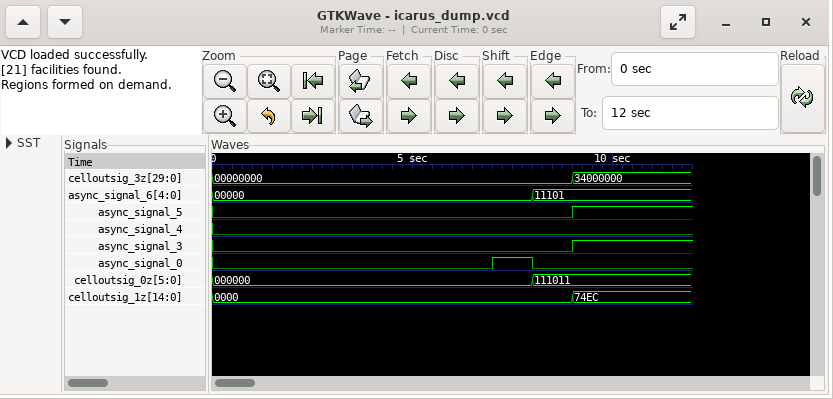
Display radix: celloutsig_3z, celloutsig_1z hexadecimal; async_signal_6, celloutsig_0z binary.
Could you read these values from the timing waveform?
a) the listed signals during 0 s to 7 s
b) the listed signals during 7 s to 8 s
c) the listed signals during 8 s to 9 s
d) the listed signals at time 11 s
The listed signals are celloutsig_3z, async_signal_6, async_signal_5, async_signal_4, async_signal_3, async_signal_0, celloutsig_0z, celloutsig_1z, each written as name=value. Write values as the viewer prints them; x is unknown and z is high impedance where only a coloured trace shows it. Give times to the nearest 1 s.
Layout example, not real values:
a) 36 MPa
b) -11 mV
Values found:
a) celloutsig_3z=00000000, async_signal_6=00000, async_signal_5=0, async_signal_4=0, async_signal_3=0, async_signal_0=0, celloutsig_0z=000000, celloutsig_1z=0000
b) celloutsig_3z=00000000, async_signal_6=00000, async_signal_5=0, async_signal_4=0, async_signal_3=0, async_signal_0=1, celloutsig_0z=000000, celloutsig_1z=0000
c) celloutsig_3z=00000000, async_signal_6=11101, async_signal_5=0, async_signal_4=0, async_signal_3=0, async_signal_0=0, celloutsig_0z=111011, celloutsig_1z=0000
d) celloutsig_3z=34000000, async_signal_6=11101, async_signal_5=1, async_signal_4=0, async_signal_3=1, async_signal_0=0, celloutsig_0z=111011, celloutsig_1z=74EC
